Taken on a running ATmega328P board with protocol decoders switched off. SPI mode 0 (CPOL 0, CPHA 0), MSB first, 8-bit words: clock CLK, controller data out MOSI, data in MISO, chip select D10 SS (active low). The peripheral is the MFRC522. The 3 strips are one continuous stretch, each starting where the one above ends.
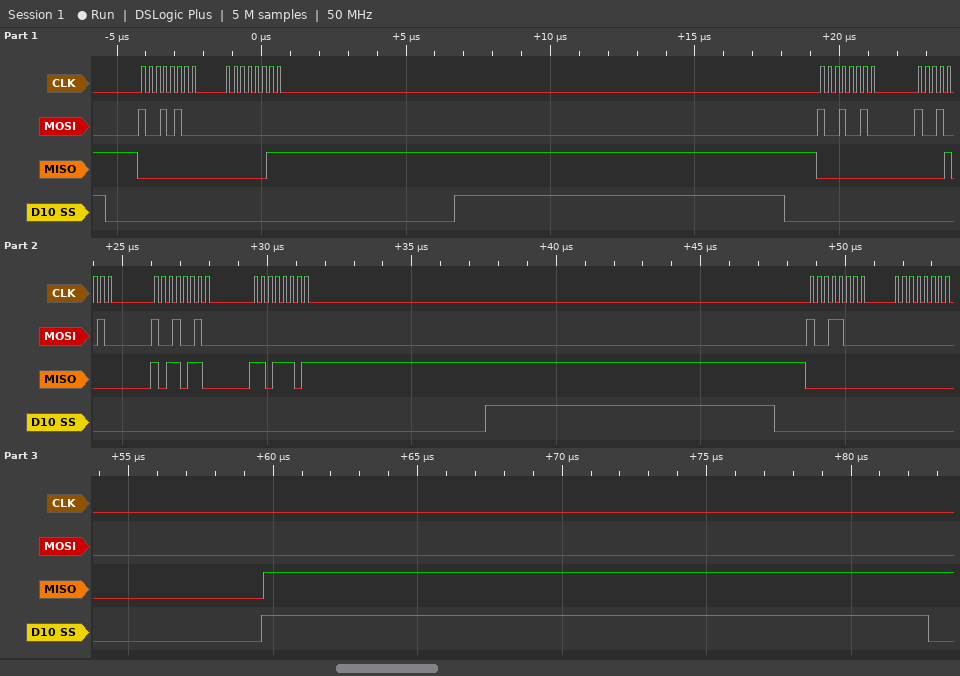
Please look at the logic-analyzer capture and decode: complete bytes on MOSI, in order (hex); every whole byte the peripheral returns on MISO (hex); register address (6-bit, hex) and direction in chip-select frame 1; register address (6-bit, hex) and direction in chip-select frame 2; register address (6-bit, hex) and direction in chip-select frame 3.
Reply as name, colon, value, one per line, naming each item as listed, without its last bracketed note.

complete bytes on MOSI, in order: 0x94 0x00 0x92 0x92 0x92 0x00 0x98 0x00
every whole byte the peripheral returns on MISO: 0x00 0x03 0x00 0x08 0xB6 0xDD 0x00 0x00
register address (6-bit, hex) and direction in chip-select frame 1: 0x0A read
register address (6-bit, hex) and direction in chip-select frame 2: 0x09 read
register address (6-bit, hex) and direction in chip-select frame 3: 0x0C read
